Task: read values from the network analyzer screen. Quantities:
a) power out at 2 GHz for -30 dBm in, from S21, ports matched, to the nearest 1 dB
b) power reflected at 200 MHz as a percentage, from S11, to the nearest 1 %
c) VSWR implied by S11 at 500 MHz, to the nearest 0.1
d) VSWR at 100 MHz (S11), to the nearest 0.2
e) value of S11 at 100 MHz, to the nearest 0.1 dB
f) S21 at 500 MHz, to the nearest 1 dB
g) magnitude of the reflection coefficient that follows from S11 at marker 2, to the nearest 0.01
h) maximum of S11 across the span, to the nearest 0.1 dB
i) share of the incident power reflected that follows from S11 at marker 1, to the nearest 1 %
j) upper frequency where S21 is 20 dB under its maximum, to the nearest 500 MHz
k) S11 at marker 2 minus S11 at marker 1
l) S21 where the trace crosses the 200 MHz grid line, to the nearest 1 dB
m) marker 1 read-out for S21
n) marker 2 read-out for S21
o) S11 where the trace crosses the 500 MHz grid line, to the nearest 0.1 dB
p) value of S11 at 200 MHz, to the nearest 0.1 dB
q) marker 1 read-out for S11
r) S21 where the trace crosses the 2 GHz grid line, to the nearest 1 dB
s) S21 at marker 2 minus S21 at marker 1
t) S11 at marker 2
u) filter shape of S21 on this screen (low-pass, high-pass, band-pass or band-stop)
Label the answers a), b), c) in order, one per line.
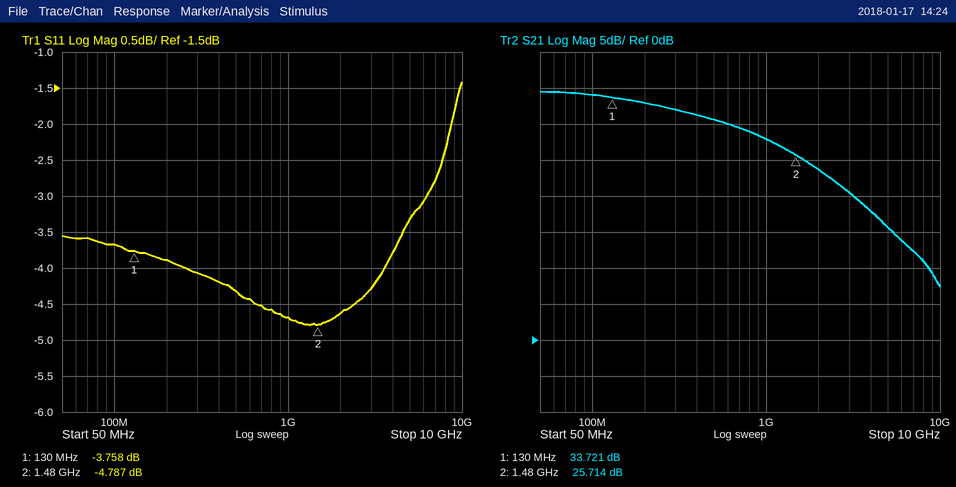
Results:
a) -6 dBm
b) 41 %
c) 4.1
d) 4.8
e) -3.7 dB
f) 31 dB
g) 0.58
h) -1.4 dB
i) 42 %
j) 5.5 GHz
k) -1.029 dB
l) 33 dB
m) 33.721 dB
n) 25.714 dB
o) -4.3 dB
p) -3.9 dB
q) -3.758 dB
r) 24 dB
s) -8.007 dB
t) -4.787 dB
u) low-pass
